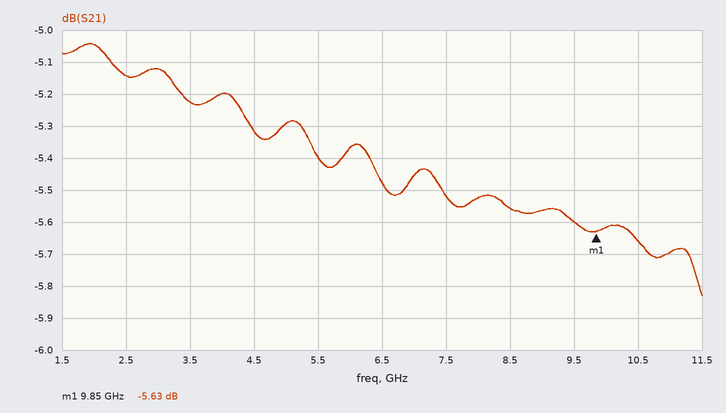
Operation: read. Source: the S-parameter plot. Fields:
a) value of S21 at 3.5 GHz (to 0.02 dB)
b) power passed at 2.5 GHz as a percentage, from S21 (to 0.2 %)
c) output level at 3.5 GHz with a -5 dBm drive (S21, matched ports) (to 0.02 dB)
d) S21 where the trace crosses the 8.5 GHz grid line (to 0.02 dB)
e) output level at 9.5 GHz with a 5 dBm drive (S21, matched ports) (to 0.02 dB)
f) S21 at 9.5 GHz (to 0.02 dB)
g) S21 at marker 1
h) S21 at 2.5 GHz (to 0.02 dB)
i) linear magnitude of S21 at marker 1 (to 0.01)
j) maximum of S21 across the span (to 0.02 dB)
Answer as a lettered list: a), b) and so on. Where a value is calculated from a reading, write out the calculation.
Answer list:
a) -5.22 dB
b) 10^(-5.14/10) ≈ 30.6 %
c) -5 dBm + (-5.22 dB) = -10.22 dBm
d) -5.56 dB
e) 5 dBm + (-5.60 dB) = -0.60 dBm
f) -5.60 dB
g) -5.63 dB
h) -5.14 dB
i) 10^(-5.63/20) ≈ 0.52
j) -5.04 dB
